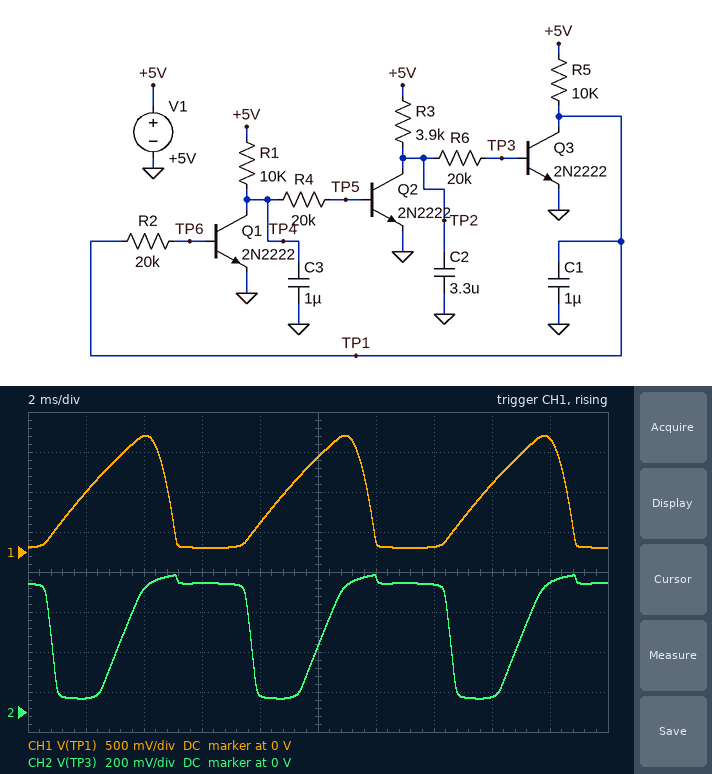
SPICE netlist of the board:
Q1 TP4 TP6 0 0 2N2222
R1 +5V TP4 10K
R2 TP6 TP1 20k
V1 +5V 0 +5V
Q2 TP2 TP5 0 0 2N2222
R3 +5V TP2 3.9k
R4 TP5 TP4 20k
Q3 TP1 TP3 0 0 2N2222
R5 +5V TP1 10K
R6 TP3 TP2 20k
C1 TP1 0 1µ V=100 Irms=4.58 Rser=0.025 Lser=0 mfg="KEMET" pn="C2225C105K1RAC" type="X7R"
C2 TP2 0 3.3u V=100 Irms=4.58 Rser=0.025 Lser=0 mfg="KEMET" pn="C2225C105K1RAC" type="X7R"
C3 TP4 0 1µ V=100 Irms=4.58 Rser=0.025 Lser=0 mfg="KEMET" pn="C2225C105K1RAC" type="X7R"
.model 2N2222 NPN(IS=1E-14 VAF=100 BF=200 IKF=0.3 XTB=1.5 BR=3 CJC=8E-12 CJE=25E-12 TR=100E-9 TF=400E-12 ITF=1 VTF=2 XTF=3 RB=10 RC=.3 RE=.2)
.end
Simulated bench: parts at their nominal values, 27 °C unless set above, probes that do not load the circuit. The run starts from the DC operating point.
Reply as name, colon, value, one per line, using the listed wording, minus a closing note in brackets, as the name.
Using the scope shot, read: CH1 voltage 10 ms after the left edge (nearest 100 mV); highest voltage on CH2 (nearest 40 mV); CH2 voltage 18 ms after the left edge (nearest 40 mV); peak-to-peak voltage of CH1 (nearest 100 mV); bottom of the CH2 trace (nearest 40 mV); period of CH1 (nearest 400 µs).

CH1 voltage 10 ms after the left edge: 1.2 V
highest voltage on CH2: 680 mV
CH2 voltage 18 ms after the left edge: 640 mV
peak-to-peak voltage of CH1: 1.4 V
bottom of the CH2 trace: 80 mV
period of CH1: 6.8 ms
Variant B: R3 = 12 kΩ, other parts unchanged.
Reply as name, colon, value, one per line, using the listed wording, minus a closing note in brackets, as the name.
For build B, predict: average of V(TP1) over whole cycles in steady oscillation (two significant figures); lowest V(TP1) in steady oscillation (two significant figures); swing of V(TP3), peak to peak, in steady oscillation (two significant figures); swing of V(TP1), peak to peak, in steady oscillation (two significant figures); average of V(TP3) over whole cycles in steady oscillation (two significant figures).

average of V(TP1) over whole cycles in steady oscillation: 1.2 V
lowest V(TP1) in steady oscillation: 67 mV
swing of V(TP3), peak to peak, in steady oscillation: 630 mV
swing of V(TP1), peak to peak, in steady oscillation: 2.2 V
average of V(TP3) over whole cycles in steady oscillation: 430 mV
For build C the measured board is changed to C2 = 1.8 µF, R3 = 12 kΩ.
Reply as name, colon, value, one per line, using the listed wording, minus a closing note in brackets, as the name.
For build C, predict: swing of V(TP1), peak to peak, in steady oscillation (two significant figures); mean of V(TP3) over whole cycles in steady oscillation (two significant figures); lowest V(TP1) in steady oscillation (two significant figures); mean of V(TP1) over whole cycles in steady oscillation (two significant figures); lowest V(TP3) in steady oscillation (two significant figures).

swing of V(TP1), peak to peak, in steady oscillation: 1.7 V
mean of V(TP3) over whole cycles in steady oscillation: 420 mV
lowest V(TP1) in steady oscillation: 59 mV
mean of V(TP1) over whole cycles in steady oscillation: 870 mV
lowest V(TP3) in steady oscillation: 45 mV
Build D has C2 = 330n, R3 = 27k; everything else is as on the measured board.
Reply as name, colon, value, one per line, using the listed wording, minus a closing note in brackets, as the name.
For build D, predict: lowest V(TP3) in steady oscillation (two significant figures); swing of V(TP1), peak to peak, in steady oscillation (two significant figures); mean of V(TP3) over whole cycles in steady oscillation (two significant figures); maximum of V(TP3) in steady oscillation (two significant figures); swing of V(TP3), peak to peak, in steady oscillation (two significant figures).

lowest V(TP3) in steady oscillation: 32 mV
swing of V(TP1), peak to peak, in steady oscillation: 1.3 V
mean of V(TP3) over whole cycles in steady oscillation: 380 mV
maximum of V(TP3) in steady oscillation: 690 mV
swing of V(TP3), peak to peak, in steady oscillation: 650 mV
